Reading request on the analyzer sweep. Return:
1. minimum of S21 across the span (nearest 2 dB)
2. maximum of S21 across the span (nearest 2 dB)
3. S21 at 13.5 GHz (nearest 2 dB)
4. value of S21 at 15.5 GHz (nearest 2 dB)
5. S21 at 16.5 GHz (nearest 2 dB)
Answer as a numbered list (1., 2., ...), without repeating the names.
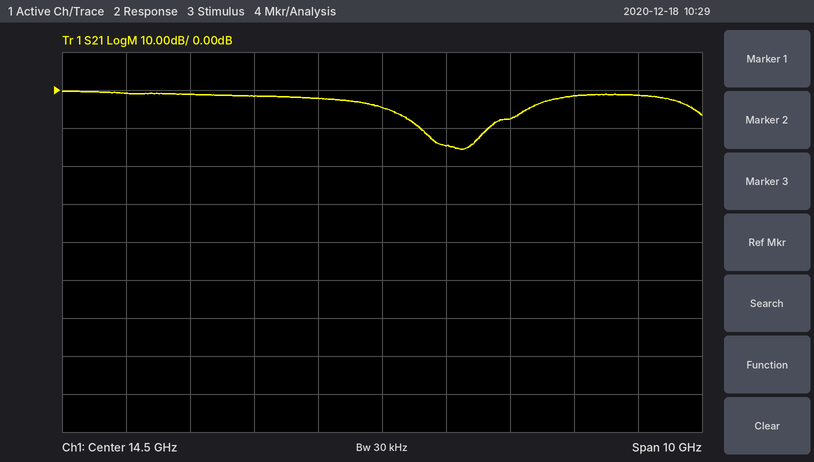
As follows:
1. -16 dB
2. 0 dB
3. -2 dB
4. -14 dB
5. -8 dB
